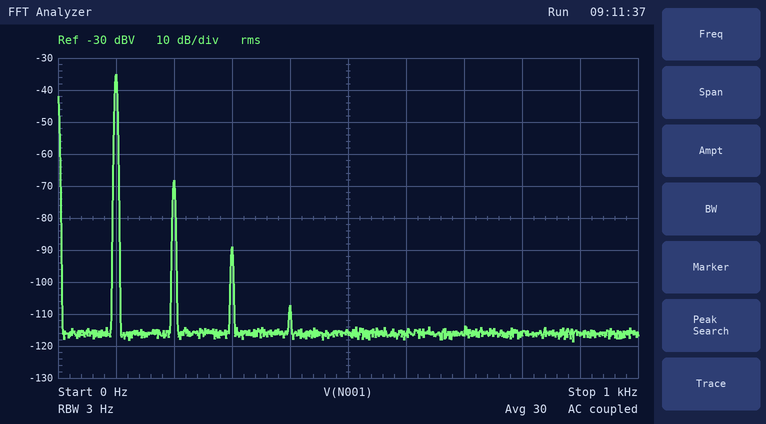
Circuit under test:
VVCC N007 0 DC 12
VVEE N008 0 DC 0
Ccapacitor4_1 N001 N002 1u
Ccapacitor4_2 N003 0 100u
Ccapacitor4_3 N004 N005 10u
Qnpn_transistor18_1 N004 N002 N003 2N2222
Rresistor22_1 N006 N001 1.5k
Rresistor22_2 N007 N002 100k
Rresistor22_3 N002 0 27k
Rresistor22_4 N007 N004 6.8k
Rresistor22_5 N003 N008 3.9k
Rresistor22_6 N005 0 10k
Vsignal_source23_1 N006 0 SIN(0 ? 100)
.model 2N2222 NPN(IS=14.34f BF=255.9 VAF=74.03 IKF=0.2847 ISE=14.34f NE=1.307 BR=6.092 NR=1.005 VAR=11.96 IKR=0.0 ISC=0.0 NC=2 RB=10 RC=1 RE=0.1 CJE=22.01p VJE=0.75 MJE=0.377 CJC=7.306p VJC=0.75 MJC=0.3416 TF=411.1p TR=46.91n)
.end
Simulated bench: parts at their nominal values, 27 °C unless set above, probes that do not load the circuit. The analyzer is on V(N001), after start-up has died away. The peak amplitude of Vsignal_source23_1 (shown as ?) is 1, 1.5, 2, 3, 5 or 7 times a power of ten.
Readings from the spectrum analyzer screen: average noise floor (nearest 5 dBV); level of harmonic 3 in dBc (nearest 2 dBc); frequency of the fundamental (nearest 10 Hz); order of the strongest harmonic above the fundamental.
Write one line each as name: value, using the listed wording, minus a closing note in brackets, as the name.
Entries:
average noise floor: -115 dBV
level of harmonic 3 in dBc: -54 dBc
frequency of the fundamental: 100 Hz
order of the strongest harmonic above the fundamental: 2
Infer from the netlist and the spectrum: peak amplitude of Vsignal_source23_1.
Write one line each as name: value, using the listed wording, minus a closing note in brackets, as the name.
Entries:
peak amplitude of Vsignal_source23_1: 30 mV
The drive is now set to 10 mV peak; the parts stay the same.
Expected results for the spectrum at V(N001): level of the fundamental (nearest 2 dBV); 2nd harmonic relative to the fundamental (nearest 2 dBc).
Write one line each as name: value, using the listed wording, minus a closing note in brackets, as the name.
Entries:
level of the fundamental: -44 dBV
2nd harmonic relative to the fundamental: -42 dBc
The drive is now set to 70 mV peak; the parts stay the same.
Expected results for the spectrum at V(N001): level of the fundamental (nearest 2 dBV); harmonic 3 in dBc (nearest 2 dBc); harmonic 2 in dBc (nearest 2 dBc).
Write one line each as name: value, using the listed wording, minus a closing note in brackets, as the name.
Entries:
level of the fundamental: -28 dBV
harmonic 3 in dBc: -42 dBc
harmonic 2 in dBc: -28 dBc
